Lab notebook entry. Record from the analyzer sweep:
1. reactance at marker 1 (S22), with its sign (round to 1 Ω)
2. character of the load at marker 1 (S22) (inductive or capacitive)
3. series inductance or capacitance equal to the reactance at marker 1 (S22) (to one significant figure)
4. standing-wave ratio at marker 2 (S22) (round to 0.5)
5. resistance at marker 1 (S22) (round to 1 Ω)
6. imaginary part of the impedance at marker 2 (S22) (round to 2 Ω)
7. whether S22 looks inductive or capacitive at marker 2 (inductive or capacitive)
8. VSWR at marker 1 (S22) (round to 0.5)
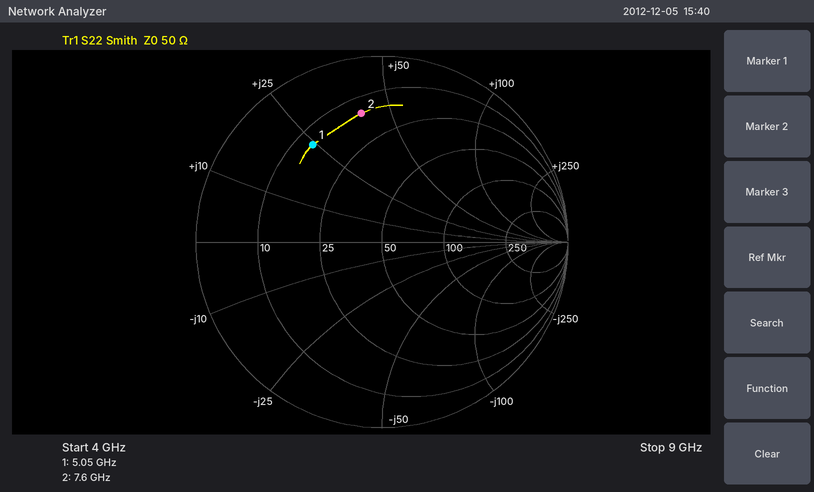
+24 Ω
inductive
800 pH
5.5
14 Ω
+40 Ω
inductive
4.5
